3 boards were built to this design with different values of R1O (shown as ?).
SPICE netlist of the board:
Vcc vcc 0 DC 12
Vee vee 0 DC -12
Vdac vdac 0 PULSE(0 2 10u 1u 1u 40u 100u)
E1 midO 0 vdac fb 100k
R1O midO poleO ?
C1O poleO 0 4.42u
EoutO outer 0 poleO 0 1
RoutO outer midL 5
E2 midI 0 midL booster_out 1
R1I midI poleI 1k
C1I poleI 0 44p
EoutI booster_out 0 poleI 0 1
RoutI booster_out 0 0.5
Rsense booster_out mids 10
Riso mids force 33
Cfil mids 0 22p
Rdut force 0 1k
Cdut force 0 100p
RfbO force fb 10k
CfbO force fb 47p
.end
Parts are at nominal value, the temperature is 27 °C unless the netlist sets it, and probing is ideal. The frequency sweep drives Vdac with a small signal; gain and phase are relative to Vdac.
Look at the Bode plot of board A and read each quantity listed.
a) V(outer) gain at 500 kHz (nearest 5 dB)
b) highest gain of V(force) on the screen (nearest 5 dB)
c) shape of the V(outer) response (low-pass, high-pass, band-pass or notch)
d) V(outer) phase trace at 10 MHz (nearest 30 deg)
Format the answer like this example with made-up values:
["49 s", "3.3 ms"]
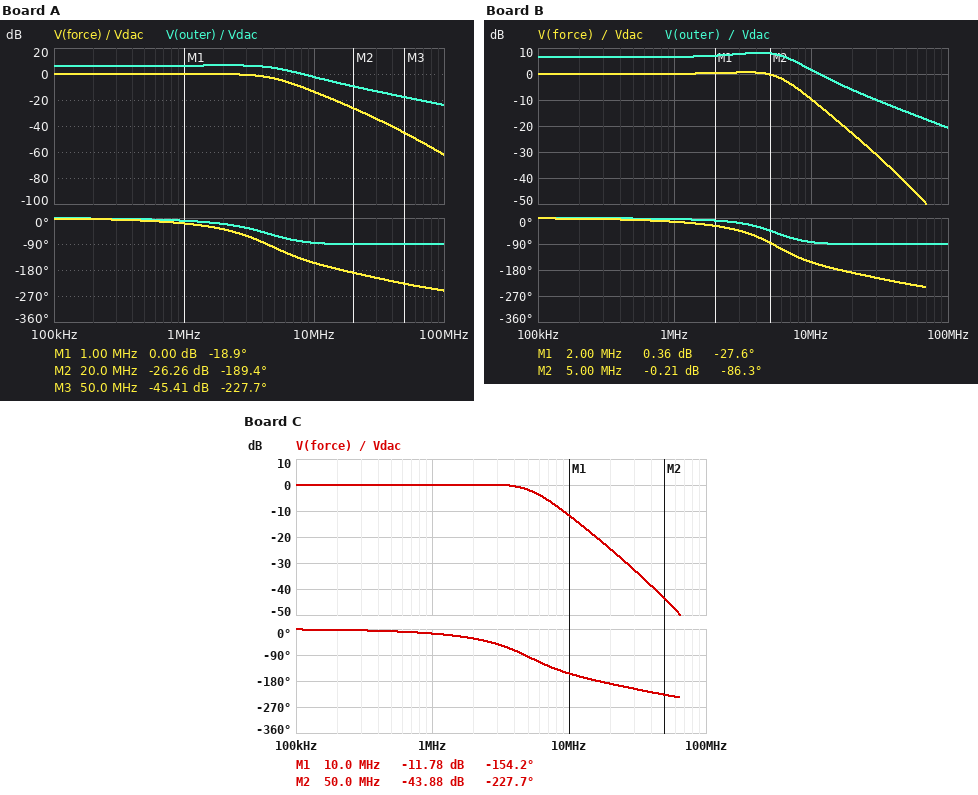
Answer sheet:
["5 dB", "0 dB", "low-pass", "-90 deg"]
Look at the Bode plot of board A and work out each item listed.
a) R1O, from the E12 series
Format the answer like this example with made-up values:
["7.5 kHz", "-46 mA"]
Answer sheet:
["560 Ω"]
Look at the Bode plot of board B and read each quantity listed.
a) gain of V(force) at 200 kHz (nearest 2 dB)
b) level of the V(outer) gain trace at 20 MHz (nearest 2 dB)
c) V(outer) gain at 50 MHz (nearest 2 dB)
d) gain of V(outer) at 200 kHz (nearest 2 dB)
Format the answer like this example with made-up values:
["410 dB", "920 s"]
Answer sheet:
["0 dB", "-6 dB", "-14 dB", "6 dB"]
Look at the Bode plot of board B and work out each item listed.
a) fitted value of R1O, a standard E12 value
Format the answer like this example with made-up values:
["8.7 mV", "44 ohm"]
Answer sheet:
["390 Ω"]
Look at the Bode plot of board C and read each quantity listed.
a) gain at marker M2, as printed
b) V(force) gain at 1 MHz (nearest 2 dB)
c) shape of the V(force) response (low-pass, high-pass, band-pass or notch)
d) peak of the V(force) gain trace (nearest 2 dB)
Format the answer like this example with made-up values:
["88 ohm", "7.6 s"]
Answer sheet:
["-43.88 dB", "0 dB", "low-pass", "0 dB"]
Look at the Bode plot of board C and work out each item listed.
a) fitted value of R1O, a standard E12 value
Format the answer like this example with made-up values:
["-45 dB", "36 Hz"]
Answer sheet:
["470 Ω"]
